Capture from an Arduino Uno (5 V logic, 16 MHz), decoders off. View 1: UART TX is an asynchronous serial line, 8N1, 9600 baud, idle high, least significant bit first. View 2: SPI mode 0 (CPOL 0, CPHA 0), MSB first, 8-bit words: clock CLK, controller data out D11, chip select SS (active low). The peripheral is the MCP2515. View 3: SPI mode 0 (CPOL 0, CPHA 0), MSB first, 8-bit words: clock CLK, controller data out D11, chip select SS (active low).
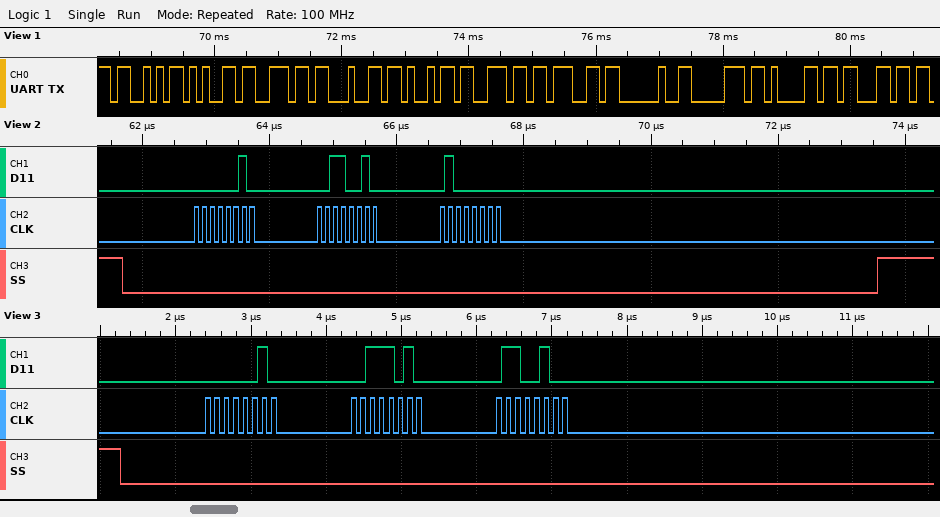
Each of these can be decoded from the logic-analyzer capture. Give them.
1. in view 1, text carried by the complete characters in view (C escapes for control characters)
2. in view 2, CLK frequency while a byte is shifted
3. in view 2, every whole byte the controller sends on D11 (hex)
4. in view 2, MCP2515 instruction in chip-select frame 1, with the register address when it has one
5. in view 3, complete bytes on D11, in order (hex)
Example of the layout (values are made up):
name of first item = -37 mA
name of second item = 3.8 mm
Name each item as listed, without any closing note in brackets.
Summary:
in view 1, text carried by the complete characters in view = "Sending pac"
in view 2, CLK frequency while a byte is shifted = 8 MHz
in view 2, every whole byte the controller sends on D11 = 02 32 40
in view 2, MCP2515 instruction in chip-select frame 1, with the register address when it has one = WRITE 0x32
in view 3, complete bytes on D11, in order = 0x02 0x3A 0x64
